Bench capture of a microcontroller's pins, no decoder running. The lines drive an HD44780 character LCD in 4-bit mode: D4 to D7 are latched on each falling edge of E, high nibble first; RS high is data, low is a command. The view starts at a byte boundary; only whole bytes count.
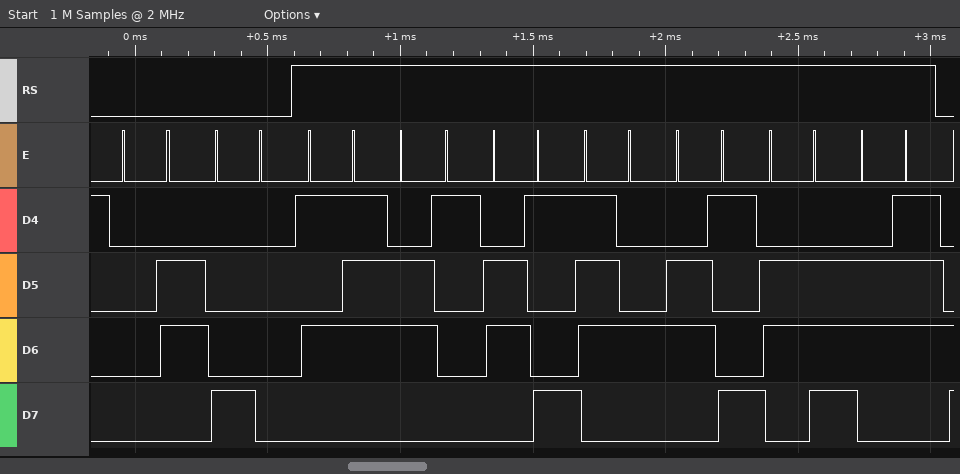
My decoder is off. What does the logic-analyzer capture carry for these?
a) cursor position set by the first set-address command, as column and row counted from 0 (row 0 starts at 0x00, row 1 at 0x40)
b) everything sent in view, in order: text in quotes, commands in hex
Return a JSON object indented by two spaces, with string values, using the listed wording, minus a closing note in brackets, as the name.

{
  "cursor position set by the first set-address command, as column and row counted from 0": "column 0, row 0",
  "everything sent in view, in order: text in quotes, commands in hex": "0x06 0x80 \"Waiting\""
}
